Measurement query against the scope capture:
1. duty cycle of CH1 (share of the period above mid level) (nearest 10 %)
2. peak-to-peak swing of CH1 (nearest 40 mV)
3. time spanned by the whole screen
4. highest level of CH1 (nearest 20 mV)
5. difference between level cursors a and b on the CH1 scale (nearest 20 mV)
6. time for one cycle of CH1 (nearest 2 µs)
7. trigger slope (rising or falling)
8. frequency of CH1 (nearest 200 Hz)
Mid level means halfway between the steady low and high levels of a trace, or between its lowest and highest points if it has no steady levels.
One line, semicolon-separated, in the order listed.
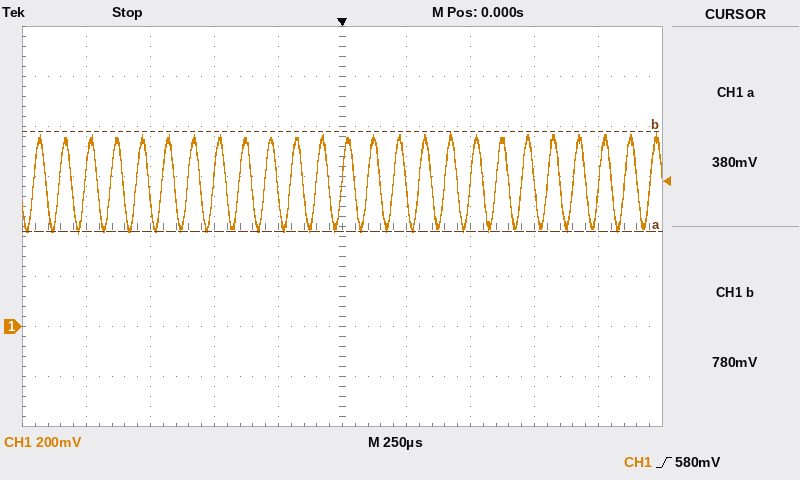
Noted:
50 %; 400 mV; 2.5 ms; 780 mV; 400 mV; 100 µs; rising; 10.0 kHz
